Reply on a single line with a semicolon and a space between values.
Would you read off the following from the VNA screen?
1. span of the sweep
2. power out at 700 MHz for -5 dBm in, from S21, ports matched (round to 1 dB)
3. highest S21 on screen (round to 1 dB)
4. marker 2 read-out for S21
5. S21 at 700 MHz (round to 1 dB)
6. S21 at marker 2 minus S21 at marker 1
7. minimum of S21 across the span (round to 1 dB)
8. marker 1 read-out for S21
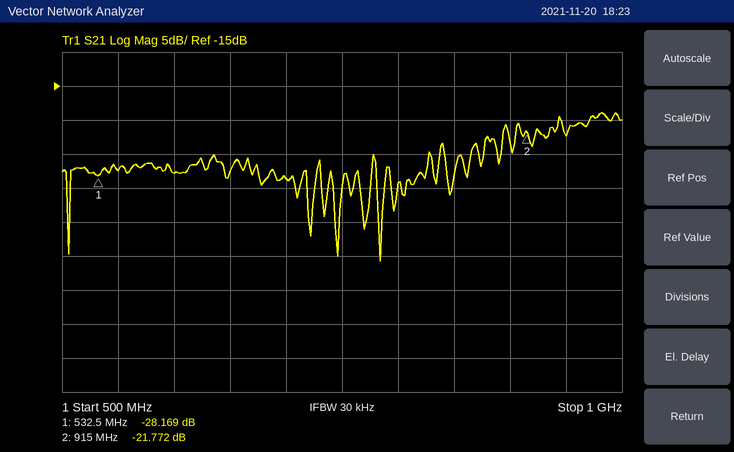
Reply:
500 MHz; -34 dBm; -19 dB; -21.772 dB; -29 dB; 6.397 dB; -41 dB; -28.169 dB
